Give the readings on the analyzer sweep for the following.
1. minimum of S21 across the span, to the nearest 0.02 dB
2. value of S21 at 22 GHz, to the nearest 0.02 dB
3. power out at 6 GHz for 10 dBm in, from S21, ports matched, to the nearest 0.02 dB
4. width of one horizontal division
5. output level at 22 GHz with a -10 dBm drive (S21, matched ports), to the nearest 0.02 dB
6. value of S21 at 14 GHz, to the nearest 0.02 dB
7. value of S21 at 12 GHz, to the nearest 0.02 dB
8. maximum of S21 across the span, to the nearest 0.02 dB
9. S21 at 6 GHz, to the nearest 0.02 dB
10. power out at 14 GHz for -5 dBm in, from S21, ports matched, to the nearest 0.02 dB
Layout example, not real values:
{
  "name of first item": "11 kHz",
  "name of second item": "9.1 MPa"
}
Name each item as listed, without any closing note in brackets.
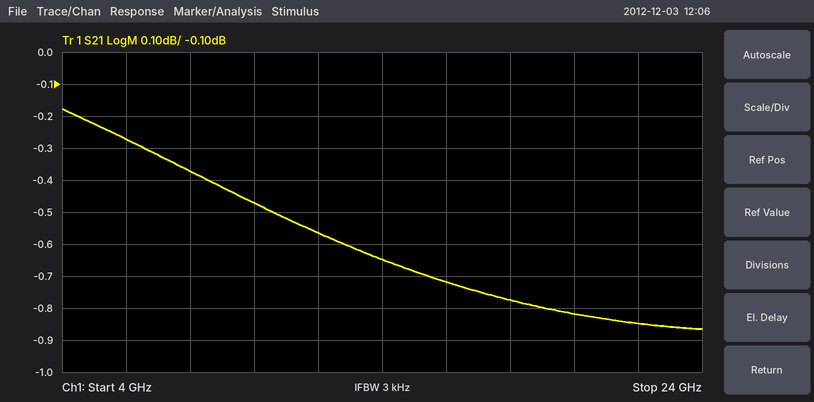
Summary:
{
  "minimum of S21 across the span, to the nearest 0.02 dB": "-0.86 dB",
  "value of S21 at 22 GHz, to the nearest 0.02 dB": "-0.84 dB",
  "power out at 6 GHz for 10 dBm in, from S21, ports matched, to the nearest 0.02 dB": "9.72 dBm",
  "width of one horizontal division": "2 GHz",
  "output level at 22 GHz with a -10 dBm drive (S21, matched ports), to the nearest 0.02 dB": "-10.84 dBm",
  "value of S21 at 14 GHz, to the nearest 0.02 dB": "-0.64 dB",
  "value of S21 at 12 GHz, to the nearest 0.02 dB": "-0.56 dB",
  "maximum of S21 across the span, to the nearest 0.02 dB": "-0.18 dB",
  "S21 at 6 GHz, to the nearest 0.02 dB": "-0.28 dB",
  "power out at 14 GHz for -5 dBm in, from S21, ports matched, to the nearest 0.02 dB": "-5.64 dBm"
}
